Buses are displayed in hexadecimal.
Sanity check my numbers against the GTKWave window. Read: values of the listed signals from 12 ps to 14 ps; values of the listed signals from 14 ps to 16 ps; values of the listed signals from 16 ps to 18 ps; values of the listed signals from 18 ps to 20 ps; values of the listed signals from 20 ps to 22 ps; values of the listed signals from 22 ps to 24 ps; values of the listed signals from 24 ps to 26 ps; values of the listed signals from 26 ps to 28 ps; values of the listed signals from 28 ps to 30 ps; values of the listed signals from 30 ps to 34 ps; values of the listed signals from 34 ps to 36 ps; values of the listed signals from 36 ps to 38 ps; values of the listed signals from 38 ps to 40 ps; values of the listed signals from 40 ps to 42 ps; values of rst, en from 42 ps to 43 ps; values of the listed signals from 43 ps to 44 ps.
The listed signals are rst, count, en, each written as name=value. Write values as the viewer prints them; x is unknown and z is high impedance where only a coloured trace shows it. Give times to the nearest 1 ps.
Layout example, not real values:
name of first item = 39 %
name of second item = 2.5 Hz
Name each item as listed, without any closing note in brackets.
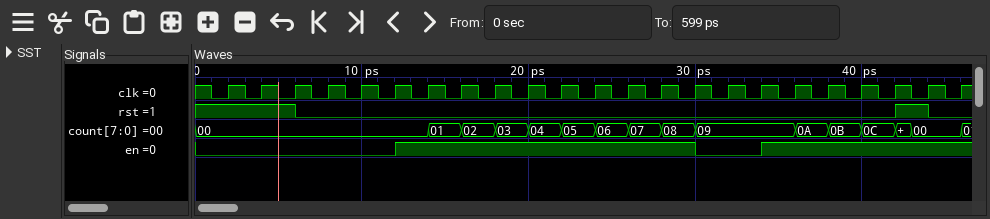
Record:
values of the listed signals from 12 ps to 14 ps = rst=0, count=00, en=1
values of the listed signals from 14 ps to 16 ps = rst=0, count=01, en=1
values of the listed signals from 16 ps to 18 ps = rst=0, count=02, en=1
values of the listed signals from 18 ps to 20 ps = rst=0, count=03, en=1
values of the listed signals from 20 ps to 22 ps = rst=0, count=04, en=1
values of the listed signals from 22 ps to 24 ps = rst=0, count=05, en=1
values of the listed signals from 24 ps to 26 ps = rst=0, count=06, en=1
values of the listed signals from 26 ps to 28 ps = rst=0, count=07, en=1
values of the listed signals from 28 ps to 30 ps = rst=0, count=08, en=1
values of the listed signals from 30 ps to 34 ps = rst=0, count=09, en=0
values of the listed signals from 34 ps to 36 ps = rst=0, count=09, en=1
values of the listed signals from 36 ps to 38 ps = rst=0, count=0A, en=1
values of the listed signals from 38 ps to 40 ps = rst=0, count=0B, en=1
values of the listed signals from 40 ps to 42 ps = rst=0, count=0C, en=1
values of rst, en from 42 ps to 43 ps = rst=1, en=1
values of the listed signals from 43 ps to 44 ps = rst=1, count=00, en=1
